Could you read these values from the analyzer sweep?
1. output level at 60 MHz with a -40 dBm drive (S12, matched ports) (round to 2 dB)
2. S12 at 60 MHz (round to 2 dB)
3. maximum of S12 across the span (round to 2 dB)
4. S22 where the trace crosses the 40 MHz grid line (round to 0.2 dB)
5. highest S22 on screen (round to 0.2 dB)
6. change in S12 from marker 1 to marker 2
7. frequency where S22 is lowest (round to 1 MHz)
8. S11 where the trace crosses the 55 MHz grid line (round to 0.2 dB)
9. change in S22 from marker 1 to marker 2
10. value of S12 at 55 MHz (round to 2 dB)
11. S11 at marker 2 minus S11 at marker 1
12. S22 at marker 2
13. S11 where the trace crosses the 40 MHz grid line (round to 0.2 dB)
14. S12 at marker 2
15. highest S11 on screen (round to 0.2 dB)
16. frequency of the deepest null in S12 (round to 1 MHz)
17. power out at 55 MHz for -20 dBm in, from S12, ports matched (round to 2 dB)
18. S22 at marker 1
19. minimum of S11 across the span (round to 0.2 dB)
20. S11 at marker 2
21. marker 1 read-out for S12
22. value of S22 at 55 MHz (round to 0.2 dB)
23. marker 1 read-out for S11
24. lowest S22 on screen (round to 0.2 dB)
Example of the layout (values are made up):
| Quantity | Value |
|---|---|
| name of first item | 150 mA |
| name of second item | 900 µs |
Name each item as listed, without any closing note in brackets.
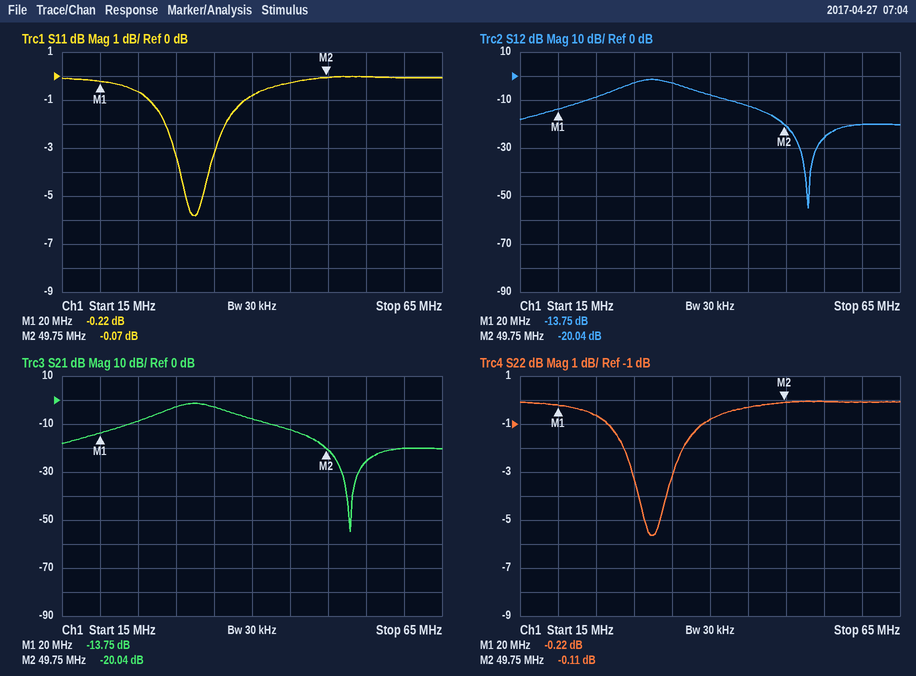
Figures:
| Quantity | Value |
|---|---|
| output level at 60 MHz with a -40 dBm drive (S12, matched ports) | -60 dBm |
| S12 at 60 MHz | -20 dB |
| maximum of S12 across the span | -2 dB |
| S22 where the trace crosses the 40 MHz grid line | -0.8 dB |
| highest S22 on screen | 0.0 dB |
| change in S12 from marker 1 to marker 2 | -6.29 dB |
| frequency where S22 is lowest | 32 MHz |
| S11 where the trace crosses the 55 MHz grid line | 0.0 dB |
| change in S22 from marker 1 to marker 2 | 0.11 dB |
| value of S12 at 55 MHz | -26 dB |
| S11 at marker 2 minus S11 at marker 1 | 0.15 dB |
| S22 at marker 2 | -0.11 dB |
| S11 where the trace crosses the 40 MHz grid line | -0.8 dB |
| S12 at marker 2 | -20.04 dB |
| highest S11 on screen | 0.0 dB |
| frequency of the deepest null in S12 | 53 MHz |
| power out at 55 MHz for -20 dBm in, from S12, ports matched | -46 dBm |
| S22 at marker 1 | -0.22 dB |
| minimum of S11 across the span | -5.8 dB |
| S11 at marker 2 | -0.07 dB |
| marker 1 read-out for S12 | -13.75 dB |
| value of S22 at 55 MHz | 0.0 dB |
| marker 1 read-out for S11 | -0.22 dB |
| lowest S22 on screen | -5.6 dB |
